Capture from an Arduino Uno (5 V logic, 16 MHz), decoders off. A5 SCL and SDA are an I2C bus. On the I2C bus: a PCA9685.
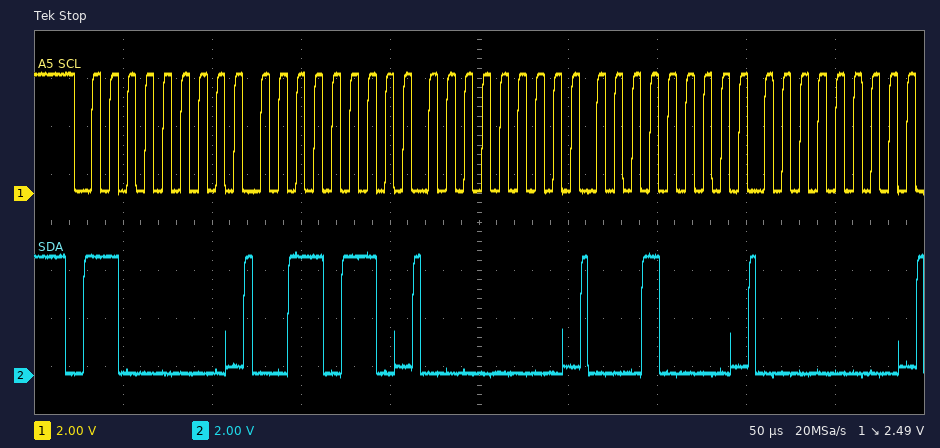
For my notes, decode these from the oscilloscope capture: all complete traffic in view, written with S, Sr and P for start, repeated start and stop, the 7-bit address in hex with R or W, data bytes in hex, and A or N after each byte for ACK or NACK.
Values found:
S 60W A 36 A 00 A 10 A 00 A
